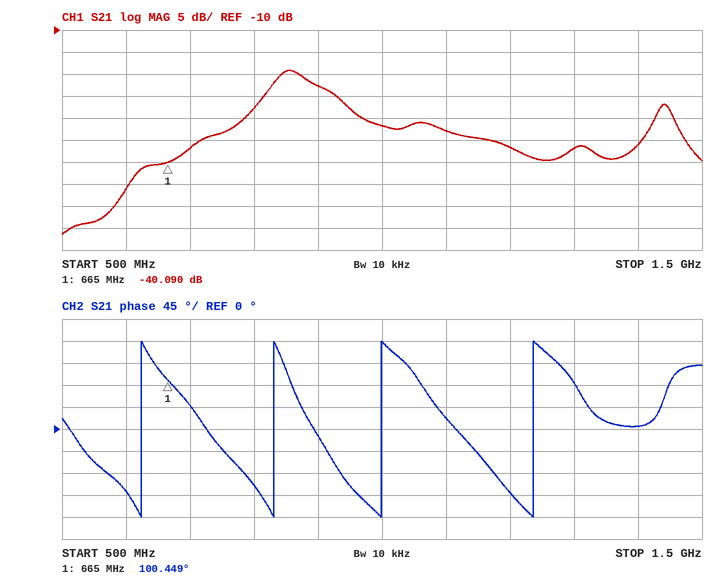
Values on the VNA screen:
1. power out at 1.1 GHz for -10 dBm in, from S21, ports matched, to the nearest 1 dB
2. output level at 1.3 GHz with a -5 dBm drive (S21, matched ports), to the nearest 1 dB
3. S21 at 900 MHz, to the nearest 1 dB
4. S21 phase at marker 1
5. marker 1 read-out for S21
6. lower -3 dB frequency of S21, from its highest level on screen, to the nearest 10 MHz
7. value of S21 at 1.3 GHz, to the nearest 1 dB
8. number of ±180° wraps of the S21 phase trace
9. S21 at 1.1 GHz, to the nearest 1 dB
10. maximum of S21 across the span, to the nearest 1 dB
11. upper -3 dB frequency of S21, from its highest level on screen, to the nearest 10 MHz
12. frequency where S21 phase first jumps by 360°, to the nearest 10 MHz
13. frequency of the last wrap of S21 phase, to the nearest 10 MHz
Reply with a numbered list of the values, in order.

1. -43 dBm
2. -42 dBm
3. -23 dB
4. 100.449°
5. -40.090 dB
6. 830 MHz
7. -37 dB
8. 4
9. -33 dB
10. -19 dB
11. 890 MHz
12. 620 MHz
13. 1.24 GHz
